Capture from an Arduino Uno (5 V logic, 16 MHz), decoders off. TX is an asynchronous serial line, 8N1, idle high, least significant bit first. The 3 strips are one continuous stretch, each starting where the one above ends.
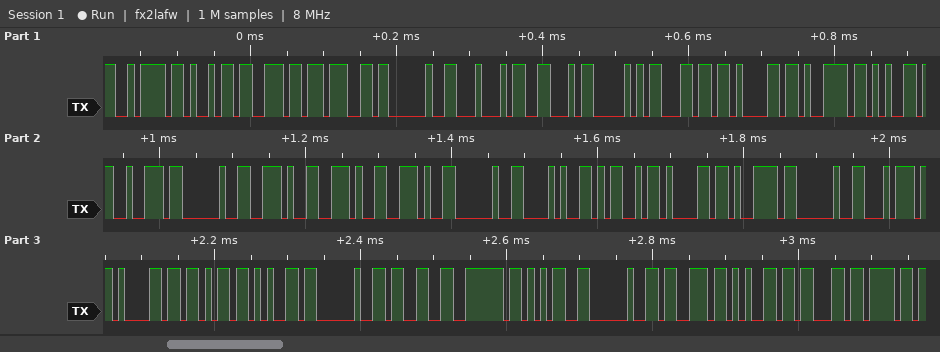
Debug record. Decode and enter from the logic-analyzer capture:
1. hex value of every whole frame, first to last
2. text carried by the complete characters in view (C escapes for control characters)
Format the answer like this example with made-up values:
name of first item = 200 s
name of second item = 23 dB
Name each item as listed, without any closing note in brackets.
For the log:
hex value of every whole frame, first to last = 7A 69 6E 67 20 44 46 50 6C 61 79 65 72 20 2E 2E 2E 20 28 4D 61 79 20 74 61 6B 65 20 33 7E 35 20 73 65 63 6F
text carried by the complete characters in view = "zing DFPlayer ... (May take 3~5 seco"
